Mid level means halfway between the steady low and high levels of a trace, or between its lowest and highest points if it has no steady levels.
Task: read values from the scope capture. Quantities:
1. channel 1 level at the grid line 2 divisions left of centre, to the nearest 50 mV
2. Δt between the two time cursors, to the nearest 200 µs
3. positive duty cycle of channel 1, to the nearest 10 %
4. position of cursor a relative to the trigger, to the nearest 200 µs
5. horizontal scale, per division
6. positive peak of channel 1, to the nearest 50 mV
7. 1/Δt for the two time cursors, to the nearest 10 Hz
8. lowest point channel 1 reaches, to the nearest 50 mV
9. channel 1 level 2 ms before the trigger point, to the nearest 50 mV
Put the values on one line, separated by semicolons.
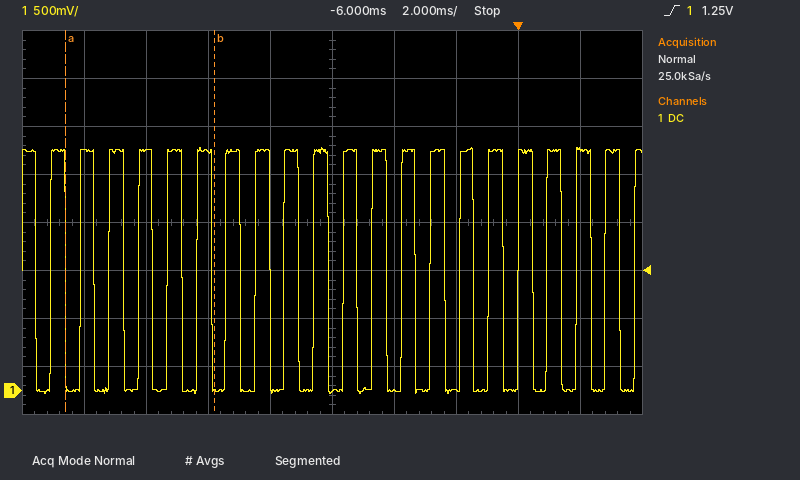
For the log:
2.50 V; 4.8 ms; 50 %; -14.6 ms; 2 ms; 2.55 V; 210 Hz; -50 mV; 0 mV
